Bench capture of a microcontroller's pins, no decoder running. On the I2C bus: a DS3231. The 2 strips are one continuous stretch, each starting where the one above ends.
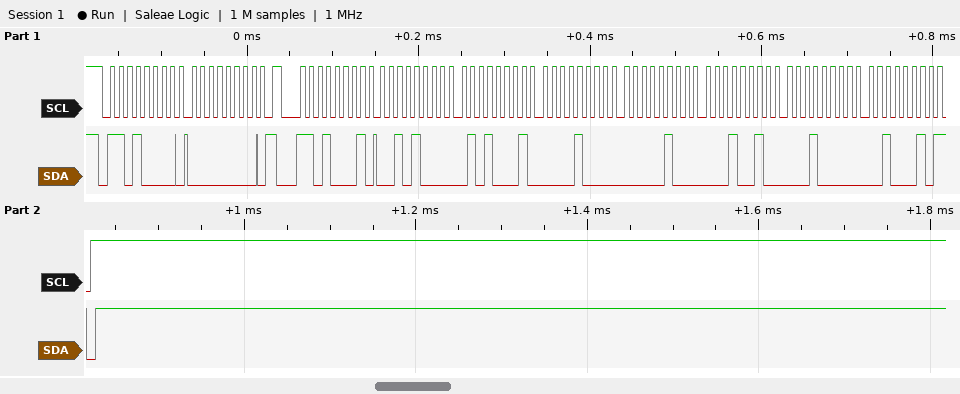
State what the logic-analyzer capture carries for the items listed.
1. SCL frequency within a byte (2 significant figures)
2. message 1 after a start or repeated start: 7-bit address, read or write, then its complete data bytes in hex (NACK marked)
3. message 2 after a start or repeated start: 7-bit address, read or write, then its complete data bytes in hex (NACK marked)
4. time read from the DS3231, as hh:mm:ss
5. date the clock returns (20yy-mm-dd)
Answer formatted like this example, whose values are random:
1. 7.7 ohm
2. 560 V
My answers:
1. 100 kHz
2. 0x68 write: 00
3. 0x68 read: 28 51 08 04 12 10 22 NACK
4. 08:51:28
5. 2022-10-12
